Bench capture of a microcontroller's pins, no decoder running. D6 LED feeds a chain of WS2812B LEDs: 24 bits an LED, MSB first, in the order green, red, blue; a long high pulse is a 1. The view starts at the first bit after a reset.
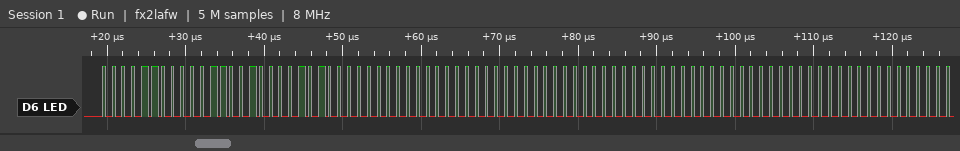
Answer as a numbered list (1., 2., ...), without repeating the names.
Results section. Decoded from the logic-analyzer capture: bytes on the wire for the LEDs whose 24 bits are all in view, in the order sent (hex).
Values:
1. 0C 19 0A 00 00 00 00 00 00
